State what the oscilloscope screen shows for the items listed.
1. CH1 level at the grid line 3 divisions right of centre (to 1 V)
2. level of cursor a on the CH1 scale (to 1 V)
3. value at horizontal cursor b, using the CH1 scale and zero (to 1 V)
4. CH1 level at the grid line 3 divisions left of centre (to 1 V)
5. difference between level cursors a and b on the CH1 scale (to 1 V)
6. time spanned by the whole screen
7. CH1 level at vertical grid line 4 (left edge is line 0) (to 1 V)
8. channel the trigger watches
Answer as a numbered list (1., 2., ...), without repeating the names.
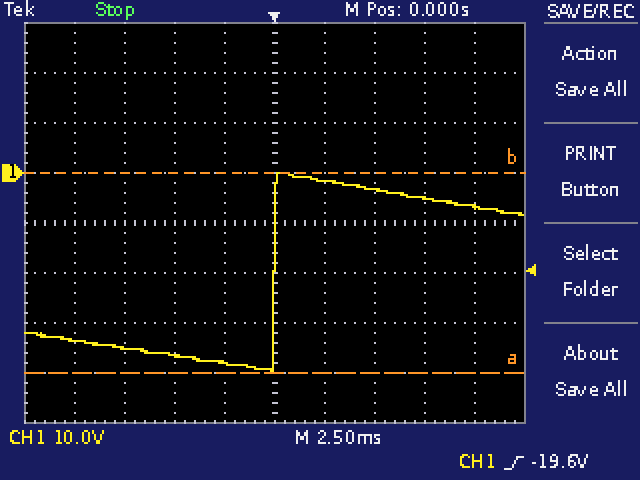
1. -5 V
2. -40 V
3. 0 V
4. -35 V
5. 40 V
6. 25 ms
7. -38 V
8. CH1
